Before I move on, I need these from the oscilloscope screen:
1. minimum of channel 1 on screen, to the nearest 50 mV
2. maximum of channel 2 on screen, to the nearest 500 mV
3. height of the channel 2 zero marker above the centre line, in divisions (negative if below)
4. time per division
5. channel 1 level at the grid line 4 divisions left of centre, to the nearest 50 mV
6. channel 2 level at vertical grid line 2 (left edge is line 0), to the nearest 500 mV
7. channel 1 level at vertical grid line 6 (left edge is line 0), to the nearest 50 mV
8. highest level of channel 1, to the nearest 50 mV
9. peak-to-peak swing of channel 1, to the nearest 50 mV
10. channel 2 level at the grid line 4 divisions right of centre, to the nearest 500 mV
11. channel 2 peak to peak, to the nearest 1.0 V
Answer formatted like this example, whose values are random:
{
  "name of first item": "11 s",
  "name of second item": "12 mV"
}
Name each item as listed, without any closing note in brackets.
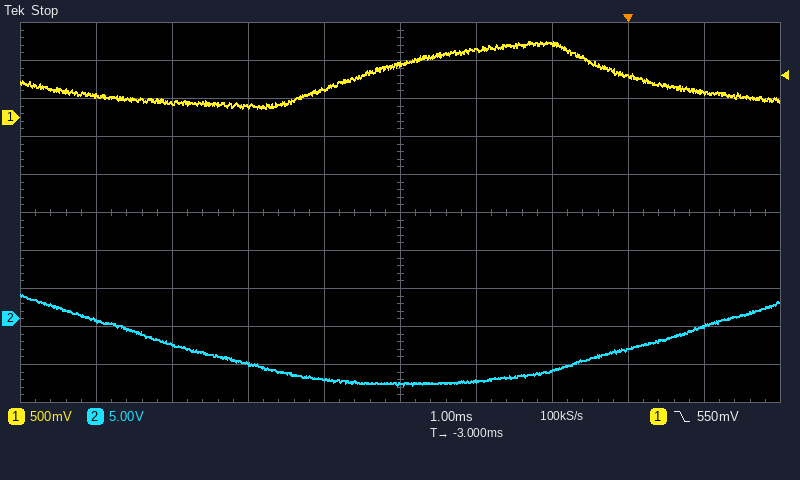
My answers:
{
  "minimum of channel 1 on screen, to the nearest 50 mV": "100 mV",
  "maximum of channel 2 on screen, to the nearest 500 mV": "3.0 V",
  "height of the channel 2 zero marker above the centre line, in divisions": "-2.8 div",
  "time per division": "1 ms",
  "channel 1 level at the grid line 4 divisions left of centre, to the nearest 50 mV": "300 mV",
  "channel 2 level at vertical grid line 2 (left edge is line 0), to the nearest 500 mV": "-3.5 V",
  "channel 1 level at vertical grid line 6 (left edge is line 0), to the nearest 50 mV": "900 mV",
  "highest level of channel 1, to the nearest 50 mV": "1.00 V",
  "peak-to-peak swing of channel 1, to the nearest 50 mV": "900 mV",
  "channel 2 level at the grid line 4 divisions right of centre, to the nearest 500 mV": "-1.0 V",
  "channel 2 peak to peak, to the nearest 1.0 V": "12.0 V"
}
